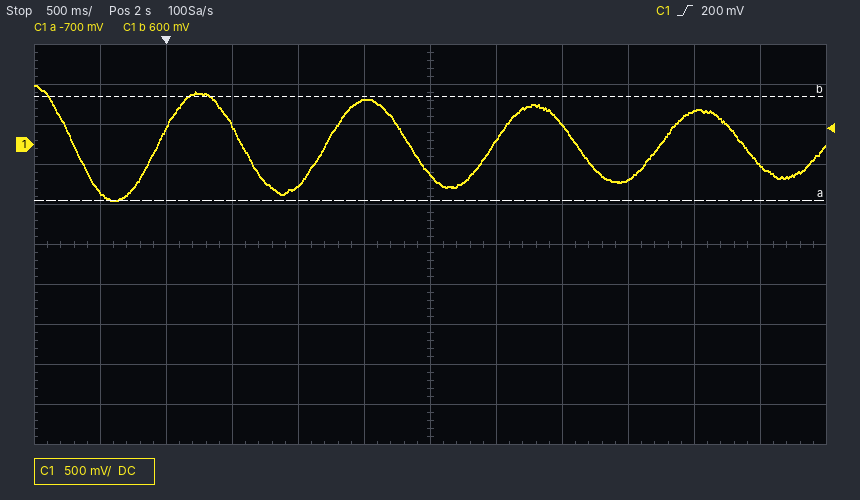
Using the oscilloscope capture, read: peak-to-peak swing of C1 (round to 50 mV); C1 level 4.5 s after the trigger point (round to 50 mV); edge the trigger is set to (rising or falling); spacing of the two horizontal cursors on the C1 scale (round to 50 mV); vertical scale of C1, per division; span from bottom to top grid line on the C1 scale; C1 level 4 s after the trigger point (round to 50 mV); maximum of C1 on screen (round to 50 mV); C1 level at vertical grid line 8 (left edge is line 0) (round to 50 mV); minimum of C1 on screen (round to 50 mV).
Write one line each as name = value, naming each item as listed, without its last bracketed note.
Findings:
peak-to-peak swing of C1 = 1.45 V
C1 level 4.5 s after the trigger point = -250 mV
edge the trigger is set to = rising
spacing of the two horizontal cursors on the C1 scale = 1.30 V
vertical scale of C1, per division = 500 mV
span from bottom to top grid line on the C1 scale = 5 V
C1 level 4 s after the trigger point = 400 mV
maximum of C1 on screen = 750 mV
C1 level at vertical grid line 8 (left edge is line 0) = 250 mV
minimum of C1 on screen = -700 mV
